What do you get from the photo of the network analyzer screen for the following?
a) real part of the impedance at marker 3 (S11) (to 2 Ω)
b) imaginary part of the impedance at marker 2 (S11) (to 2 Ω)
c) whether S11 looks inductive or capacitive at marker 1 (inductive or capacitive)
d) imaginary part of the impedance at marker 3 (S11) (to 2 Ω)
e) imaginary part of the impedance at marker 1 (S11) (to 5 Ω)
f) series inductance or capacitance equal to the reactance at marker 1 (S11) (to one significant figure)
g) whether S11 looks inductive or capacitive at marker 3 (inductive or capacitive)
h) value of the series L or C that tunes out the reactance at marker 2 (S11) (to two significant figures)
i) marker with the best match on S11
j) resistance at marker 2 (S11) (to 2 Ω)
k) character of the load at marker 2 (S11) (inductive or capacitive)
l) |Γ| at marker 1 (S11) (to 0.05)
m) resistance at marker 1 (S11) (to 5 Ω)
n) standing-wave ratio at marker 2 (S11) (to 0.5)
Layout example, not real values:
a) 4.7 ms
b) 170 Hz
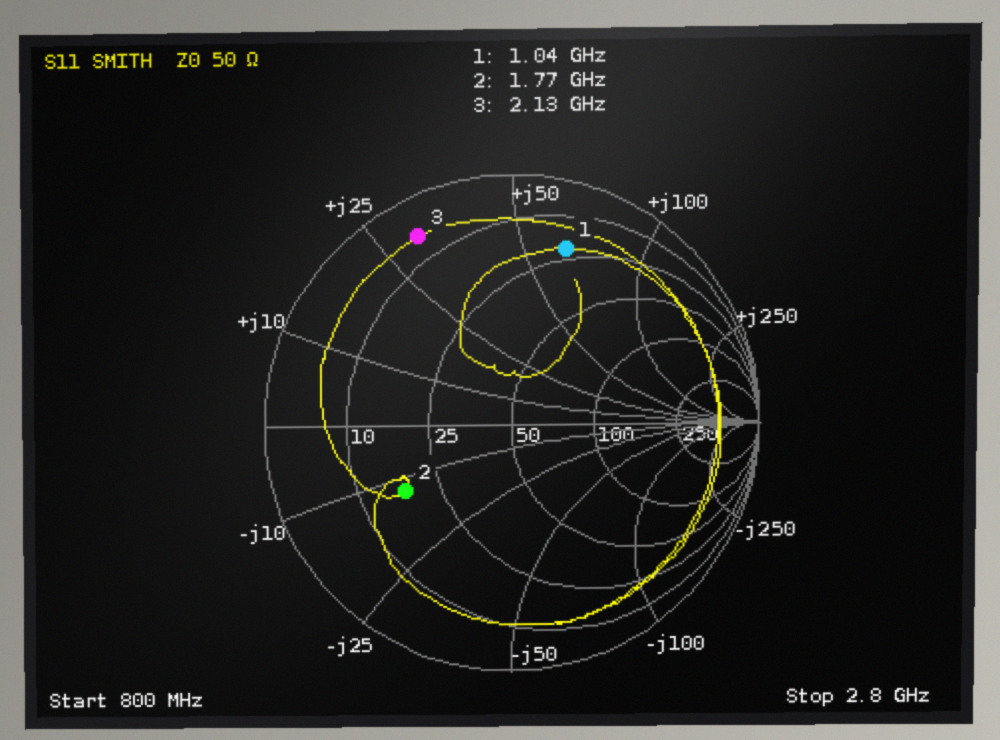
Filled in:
a) 6 Ω
b) -12 Ω
c) inductive
d) +30 Ω
e) +65 Ω
f) 10 nH
g) inductive
h) 1.1 nH
i) marker 2
j) 18 Ω
k) capacitive
l) 0.75
m) 20 Ω
n) 3.0
